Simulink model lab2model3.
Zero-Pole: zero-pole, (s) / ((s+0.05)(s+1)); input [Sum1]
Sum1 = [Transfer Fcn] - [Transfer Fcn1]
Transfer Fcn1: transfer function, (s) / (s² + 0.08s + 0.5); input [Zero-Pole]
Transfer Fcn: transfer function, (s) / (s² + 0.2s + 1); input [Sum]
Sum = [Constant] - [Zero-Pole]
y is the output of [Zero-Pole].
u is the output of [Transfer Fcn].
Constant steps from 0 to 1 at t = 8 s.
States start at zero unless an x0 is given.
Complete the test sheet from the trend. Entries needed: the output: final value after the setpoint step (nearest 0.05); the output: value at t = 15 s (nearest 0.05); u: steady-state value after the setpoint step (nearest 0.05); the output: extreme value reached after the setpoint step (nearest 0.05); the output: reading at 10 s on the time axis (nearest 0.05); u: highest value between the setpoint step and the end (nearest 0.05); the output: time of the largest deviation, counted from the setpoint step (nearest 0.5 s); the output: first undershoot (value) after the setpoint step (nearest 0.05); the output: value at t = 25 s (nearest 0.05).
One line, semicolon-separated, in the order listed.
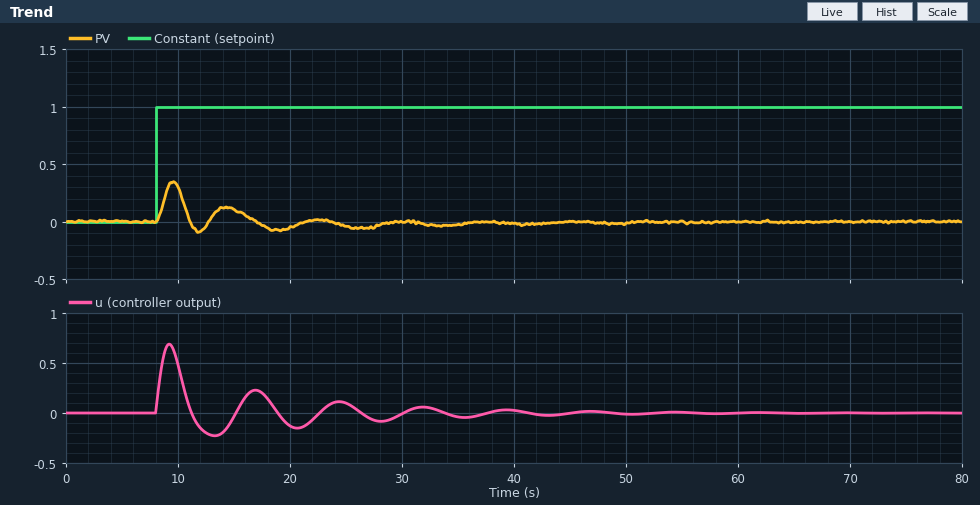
0.00; 0.10; 0.00; 0.35; 0.30; 0.70; 1.5 s; -0.10; -0.05
